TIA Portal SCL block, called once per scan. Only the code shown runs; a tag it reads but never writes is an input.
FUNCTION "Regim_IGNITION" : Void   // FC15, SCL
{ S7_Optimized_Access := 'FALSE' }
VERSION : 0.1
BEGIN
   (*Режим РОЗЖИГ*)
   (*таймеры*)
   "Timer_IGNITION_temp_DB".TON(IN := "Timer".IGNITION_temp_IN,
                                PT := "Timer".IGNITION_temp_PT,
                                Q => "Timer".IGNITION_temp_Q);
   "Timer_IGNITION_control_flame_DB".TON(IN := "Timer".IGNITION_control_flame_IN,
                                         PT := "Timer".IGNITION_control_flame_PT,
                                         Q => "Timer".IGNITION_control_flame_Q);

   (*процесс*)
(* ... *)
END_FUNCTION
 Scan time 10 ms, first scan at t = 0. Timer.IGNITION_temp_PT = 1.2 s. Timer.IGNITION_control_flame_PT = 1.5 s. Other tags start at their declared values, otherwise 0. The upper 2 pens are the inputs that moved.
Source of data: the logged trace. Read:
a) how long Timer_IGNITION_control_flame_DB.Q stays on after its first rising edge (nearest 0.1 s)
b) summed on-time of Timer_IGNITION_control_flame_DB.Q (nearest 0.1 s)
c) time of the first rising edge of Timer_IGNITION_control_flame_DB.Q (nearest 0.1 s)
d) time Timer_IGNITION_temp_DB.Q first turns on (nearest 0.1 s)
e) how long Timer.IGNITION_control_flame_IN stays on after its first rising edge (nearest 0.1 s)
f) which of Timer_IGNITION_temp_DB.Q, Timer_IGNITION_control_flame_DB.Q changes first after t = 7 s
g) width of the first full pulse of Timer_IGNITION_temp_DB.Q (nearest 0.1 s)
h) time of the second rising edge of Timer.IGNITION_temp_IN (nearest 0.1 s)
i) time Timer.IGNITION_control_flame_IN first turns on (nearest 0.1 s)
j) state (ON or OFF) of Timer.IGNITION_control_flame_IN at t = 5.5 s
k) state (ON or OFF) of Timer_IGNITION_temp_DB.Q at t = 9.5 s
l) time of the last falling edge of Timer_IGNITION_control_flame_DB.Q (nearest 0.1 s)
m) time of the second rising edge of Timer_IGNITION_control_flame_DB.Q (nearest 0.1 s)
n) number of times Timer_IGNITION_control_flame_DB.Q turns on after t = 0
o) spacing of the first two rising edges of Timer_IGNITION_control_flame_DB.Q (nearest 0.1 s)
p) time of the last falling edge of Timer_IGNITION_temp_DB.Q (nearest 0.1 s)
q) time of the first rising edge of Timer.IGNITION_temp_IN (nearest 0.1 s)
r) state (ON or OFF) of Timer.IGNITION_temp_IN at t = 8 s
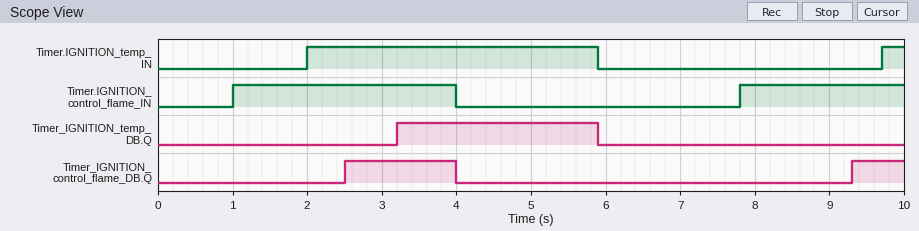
1.5 s
2.2 s
2.5 s
3.2 s
3.0 s
Timer_IGNITION_control_flame_DB.Q
2.7 s
9.7 s
1.0 s
OFF
OFF
4.0 s
9.3 s
2
6.8 s
5.9 s
2.0 s
OFF
